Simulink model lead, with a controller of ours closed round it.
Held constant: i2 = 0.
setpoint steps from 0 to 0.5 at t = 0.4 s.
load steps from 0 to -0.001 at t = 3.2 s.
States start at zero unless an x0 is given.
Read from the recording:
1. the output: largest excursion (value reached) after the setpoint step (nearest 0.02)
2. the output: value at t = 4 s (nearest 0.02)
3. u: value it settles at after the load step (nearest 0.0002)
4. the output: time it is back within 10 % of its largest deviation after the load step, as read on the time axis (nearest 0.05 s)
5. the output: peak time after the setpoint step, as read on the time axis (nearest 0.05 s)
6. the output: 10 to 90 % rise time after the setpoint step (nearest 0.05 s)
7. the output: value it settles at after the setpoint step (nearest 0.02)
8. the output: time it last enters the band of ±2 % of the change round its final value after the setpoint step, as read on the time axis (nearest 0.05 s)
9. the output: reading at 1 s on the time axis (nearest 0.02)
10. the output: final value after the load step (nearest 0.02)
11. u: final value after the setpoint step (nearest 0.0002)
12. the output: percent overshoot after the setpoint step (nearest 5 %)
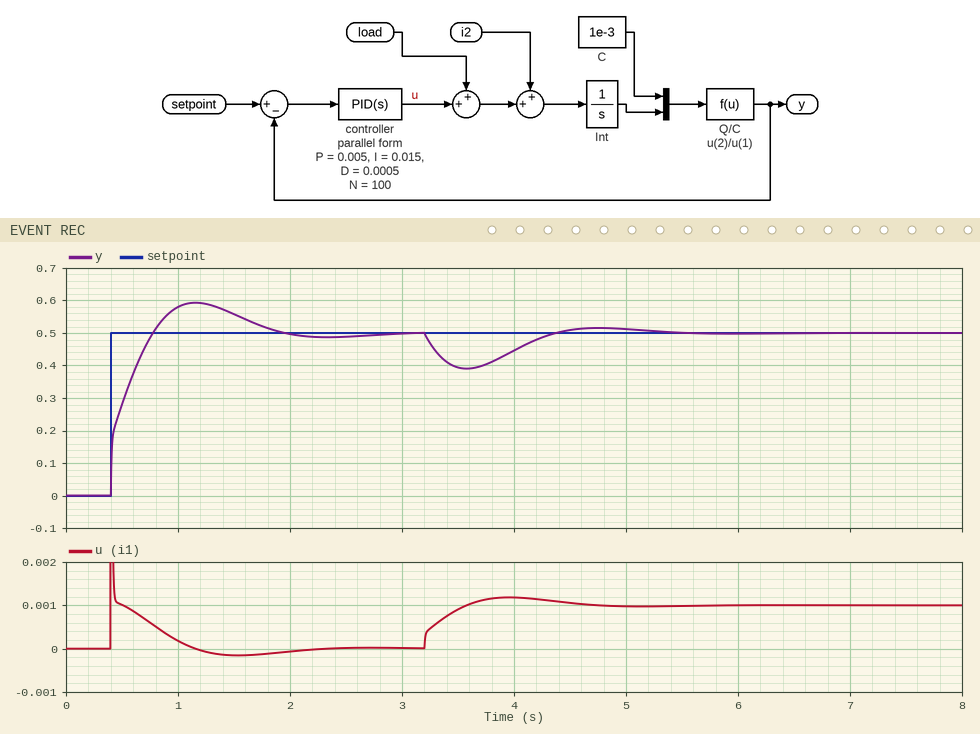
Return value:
0.60
0.44
0.0010
5.05 s
1.15 s
0.30 s
0.50
2.60 s
0.58
0.50
0.0000
20 %
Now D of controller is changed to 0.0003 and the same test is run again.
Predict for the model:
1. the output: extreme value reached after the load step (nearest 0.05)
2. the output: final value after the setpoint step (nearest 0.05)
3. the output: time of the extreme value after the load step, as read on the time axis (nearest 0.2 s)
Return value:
0.40
0.50
3.6 s
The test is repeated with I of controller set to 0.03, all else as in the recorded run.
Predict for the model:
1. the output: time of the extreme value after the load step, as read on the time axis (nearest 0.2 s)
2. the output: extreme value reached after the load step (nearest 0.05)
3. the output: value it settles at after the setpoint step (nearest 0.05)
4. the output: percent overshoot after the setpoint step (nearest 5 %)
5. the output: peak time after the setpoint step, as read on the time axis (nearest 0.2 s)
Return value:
3.4 s
0.40
0.50
25 %
1.0 s
